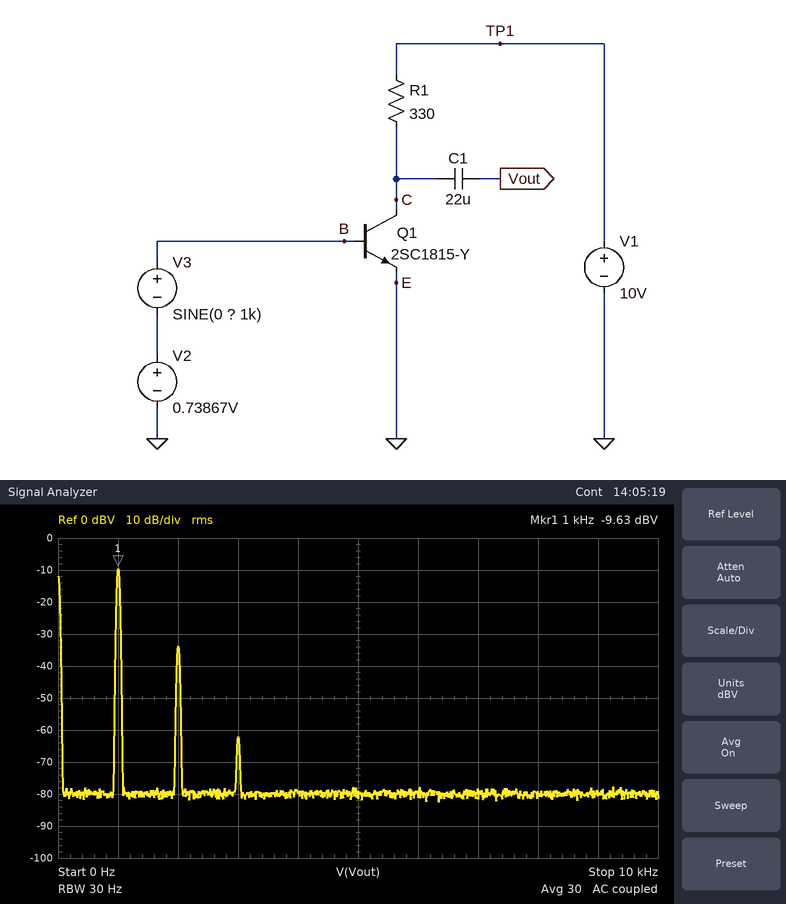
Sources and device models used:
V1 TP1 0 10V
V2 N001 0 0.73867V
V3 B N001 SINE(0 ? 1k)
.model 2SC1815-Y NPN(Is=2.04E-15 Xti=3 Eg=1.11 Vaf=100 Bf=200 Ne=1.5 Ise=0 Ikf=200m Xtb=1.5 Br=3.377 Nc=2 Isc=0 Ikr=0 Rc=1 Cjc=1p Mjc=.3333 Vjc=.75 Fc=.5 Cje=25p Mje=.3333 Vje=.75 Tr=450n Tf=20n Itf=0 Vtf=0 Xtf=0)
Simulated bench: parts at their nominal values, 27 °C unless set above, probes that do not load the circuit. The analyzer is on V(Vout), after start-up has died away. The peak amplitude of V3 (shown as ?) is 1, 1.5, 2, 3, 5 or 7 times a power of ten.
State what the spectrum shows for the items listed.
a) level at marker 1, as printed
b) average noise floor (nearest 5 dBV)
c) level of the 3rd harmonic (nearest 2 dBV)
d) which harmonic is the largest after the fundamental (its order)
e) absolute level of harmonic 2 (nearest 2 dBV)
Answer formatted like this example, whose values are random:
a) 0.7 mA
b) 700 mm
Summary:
a) -9.63 dBV
b) -80 dBV
c) -62 dBV
d) 2
e) -34 dBV
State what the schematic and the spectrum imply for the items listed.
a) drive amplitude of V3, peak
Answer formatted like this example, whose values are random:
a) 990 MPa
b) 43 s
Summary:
a) 7 mV
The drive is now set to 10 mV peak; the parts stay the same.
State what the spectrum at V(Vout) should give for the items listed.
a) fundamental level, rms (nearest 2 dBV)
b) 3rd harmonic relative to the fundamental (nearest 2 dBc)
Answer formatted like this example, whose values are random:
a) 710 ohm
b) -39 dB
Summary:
a) -6 dBV
b) -46 dBc
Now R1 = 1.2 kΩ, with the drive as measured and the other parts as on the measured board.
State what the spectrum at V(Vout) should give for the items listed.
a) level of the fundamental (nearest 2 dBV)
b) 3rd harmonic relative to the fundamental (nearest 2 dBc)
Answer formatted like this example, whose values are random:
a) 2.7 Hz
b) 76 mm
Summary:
a) 0 dBV
b) -56 dBc
